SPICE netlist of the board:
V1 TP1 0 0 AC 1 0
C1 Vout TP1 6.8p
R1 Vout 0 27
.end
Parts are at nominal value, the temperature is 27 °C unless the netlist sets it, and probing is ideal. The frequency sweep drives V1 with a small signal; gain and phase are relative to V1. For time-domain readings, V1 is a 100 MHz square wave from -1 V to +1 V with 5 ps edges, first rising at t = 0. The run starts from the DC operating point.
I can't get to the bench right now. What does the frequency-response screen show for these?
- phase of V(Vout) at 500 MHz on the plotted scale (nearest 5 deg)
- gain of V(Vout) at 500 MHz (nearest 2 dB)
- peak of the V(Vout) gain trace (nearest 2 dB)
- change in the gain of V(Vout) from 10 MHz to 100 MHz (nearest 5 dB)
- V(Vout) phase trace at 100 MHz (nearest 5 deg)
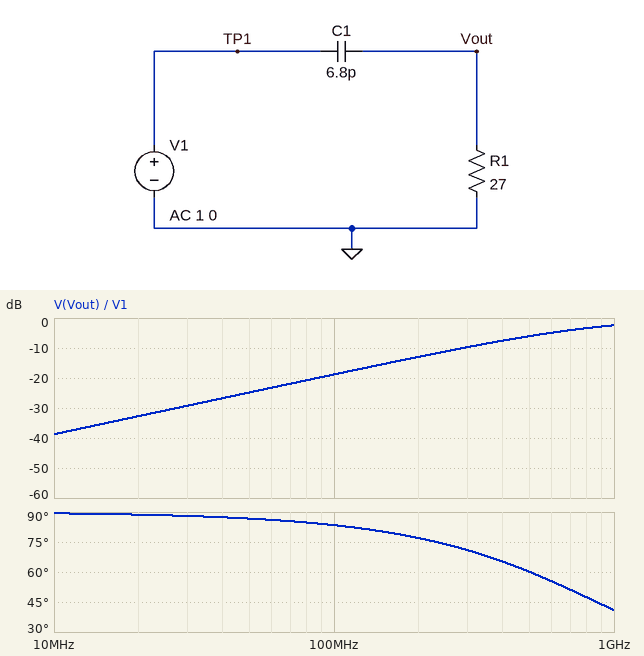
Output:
60 deg
-6 dB
-2 dB
20 dB
85 deg
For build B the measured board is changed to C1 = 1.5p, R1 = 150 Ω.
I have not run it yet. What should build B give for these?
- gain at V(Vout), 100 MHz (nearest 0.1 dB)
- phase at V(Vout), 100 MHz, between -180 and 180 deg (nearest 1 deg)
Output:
-17.1 dB
82 deg
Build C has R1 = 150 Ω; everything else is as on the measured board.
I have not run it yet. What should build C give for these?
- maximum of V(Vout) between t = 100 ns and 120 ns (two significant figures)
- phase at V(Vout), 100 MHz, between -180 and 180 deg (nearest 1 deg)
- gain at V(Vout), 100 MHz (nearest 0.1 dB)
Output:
2.0 V
57 deg
-5.4 dB
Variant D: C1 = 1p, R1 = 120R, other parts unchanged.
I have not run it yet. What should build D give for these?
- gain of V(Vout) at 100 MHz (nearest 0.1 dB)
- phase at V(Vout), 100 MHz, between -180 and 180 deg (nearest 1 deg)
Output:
-22.5 dB
86 deg
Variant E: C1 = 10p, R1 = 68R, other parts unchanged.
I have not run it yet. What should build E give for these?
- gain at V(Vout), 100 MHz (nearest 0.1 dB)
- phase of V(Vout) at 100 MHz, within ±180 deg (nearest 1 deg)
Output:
-8.1 dB
67 deg
